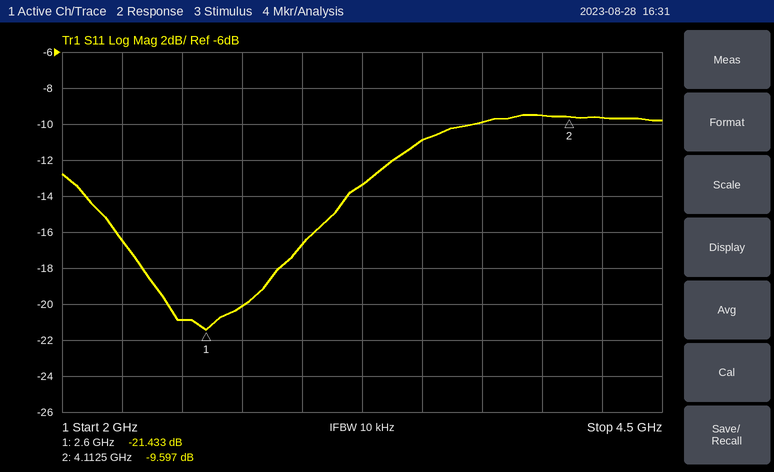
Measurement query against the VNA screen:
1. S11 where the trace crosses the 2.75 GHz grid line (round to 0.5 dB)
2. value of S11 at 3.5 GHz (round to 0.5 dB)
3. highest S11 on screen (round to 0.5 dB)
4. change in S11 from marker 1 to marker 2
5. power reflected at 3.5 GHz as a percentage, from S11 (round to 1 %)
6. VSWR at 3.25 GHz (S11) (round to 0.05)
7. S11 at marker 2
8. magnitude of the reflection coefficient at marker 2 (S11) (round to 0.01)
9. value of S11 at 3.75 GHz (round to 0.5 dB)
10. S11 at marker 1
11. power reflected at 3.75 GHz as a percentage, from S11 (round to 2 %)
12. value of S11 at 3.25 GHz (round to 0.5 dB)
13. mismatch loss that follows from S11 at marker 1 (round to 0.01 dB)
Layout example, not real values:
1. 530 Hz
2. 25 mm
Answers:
1. -20.0 dB
2. -11.0 dB
3. -9.5 dB
4. 11.836 dB
5. 8 %
6. 1.55
7. -9.597 dB
8. 0.33
9. -10.0 dB
10. -21.433 dB
11. 10 %
12. -13.5 dB
13. 0.03 dB
